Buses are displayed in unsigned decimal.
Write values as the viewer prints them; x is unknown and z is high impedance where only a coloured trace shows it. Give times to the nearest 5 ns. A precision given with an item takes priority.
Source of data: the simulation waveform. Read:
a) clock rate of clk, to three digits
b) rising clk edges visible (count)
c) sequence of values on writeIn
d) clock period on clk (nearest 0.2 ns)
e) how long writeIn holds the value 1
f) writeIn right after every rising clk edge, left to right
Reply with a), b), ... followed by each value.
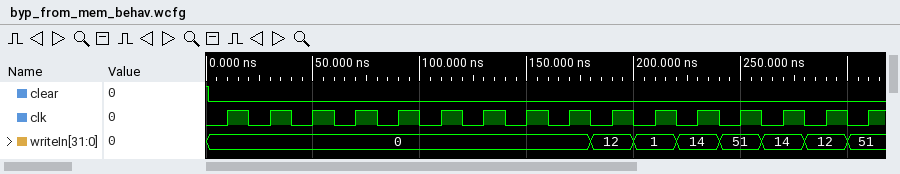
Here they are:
a) 50.0 MHz
b) 16
c) 0, 12, 1, 14, 51, 14, 12, 51
d) 20 ns
e) 20 ns
f) 0, 0, 0, 0, 0, 0, 0, 0, 0, 12, 1, 14, 51, 14, 12, 51
